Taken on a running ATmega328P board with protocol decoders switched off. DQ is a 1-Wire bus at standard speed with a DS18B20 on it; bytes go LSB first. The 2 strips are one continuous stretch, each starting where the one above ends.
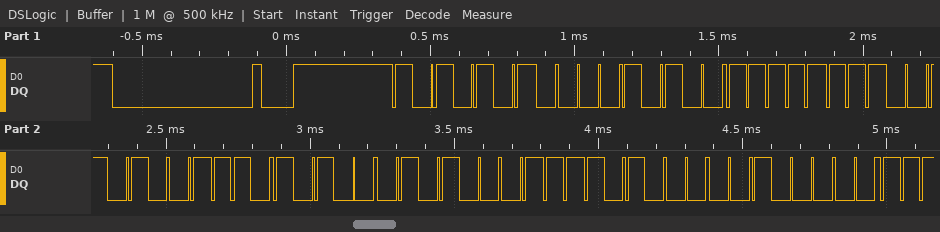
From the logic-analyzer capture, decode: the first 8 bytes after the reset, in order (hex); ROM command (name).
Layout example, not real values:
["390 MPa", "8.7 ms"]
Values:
["55 28 FF 94 2B 8A 17 04", "Match ROM"]
